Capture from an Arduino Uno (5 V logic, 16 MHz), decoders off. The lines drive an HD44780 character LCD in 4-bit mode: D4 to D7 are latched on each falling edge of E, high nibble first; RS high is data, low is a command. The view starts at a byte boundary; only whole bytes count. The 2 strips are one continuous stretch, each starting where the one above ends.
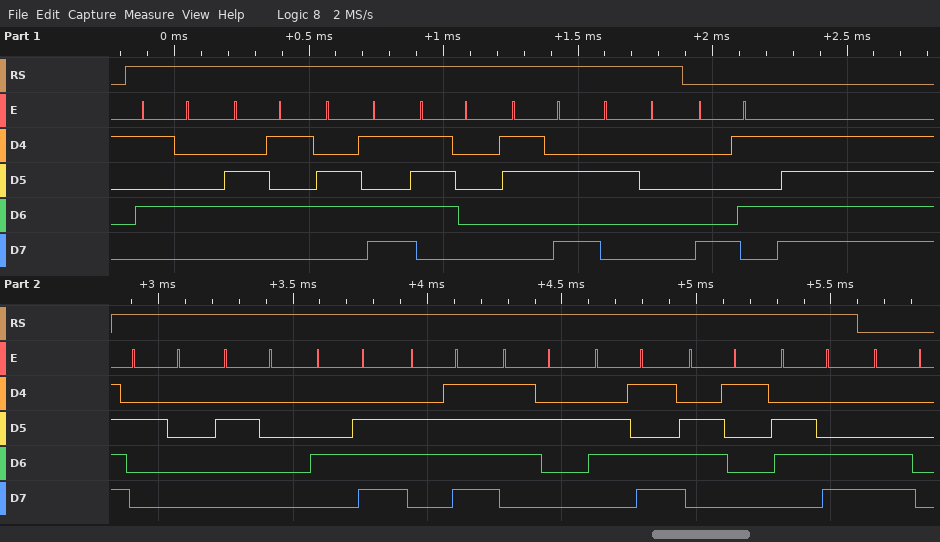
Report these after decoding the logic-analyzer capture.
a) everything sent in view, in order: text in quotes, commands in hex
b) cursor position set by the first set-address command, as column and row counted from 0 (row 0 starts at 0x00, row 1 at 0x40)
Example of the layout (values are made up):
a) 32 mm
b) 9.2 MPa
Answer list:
a) "Temp: " 0x85 "  Normal" 0xC0
b) column 5, row 0
